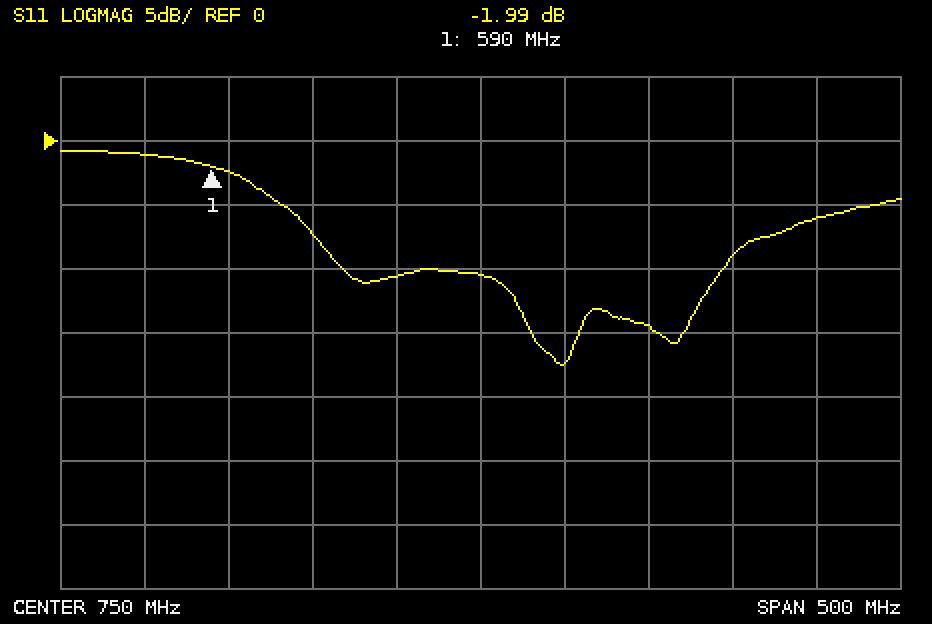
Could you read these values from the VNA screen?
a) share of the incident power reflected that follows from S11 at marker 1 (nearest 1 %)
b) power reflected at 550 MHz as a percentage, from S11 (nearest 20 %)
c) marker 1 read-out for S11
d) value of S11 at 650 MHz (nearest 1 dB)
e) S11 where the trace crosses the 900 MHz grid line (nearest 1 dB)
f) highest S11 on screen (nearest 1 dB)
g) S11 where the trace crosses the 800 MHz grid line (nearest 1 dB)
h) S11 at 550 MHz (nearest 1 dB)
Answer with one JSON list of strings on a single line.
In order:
["63 %", "80 %", "-1.99 dB", "-7 dB", "-9 dB", "-1 dB", "-17 dB", "-1 dB"]
